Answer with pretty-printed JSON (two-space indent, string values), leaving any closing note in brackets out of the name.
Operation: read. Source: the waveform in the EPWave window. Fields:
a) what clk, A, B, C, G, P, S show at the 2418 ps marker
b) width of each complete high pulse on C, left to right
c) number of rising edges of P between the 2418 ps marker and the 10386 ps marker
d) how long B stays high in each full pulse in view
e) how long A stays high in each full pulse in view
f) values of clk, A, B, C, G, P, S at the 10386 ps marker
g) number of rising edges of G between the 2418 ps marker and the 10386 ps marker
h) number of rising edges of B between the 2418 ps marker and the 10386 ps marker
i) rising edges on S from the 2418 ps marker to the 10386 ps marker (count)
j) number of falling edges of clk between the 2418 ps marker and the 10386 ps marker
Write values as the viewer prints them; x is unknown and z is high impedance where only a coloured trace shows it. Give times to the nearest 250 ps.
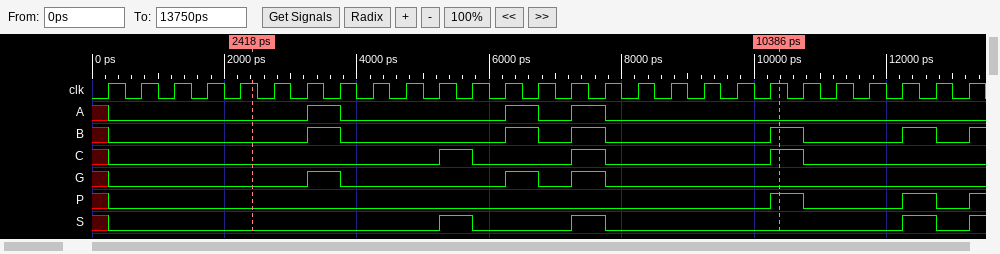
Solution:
{
  "what clk, A, B, C, G, P, S show at the 2418 ps marker": "clk=1, A=0, B=0, C=0, G=0, P=0, S=0",
  "width of each complete high pulse on C, left to right": "500 ps, 500 ps, 500 ps",
  "number of rising edges of P between the 2418 ps marker and the 10386 ps marker": "1",
  "how long B stays high in each full pulse in view": "500 ps, 500 ps, 500 ps, 500 ps, 500 ps",
  "how long A stays high in each full pulse in view": "500 ps, 500 ps, 500 ps",
  "values of clk, A, B, C, G, P, S at the 10386 ps marker": "clk=1, A=0, B=1, C=1, G=0, P=1, S=0",
  "number of rising edges of G between the 2418 ps marker and the 10386 ps marker": "3",
  "number of rising edges of B between the 2418 ps marker and the 10386 ps marker": "4",
  "rising edges on S from the 2418 ps marker to the 10386 ps marker": "2",
  "number of falling edges of clk between the 2418 ps marker and the 10386 ps marker": "16"
}
